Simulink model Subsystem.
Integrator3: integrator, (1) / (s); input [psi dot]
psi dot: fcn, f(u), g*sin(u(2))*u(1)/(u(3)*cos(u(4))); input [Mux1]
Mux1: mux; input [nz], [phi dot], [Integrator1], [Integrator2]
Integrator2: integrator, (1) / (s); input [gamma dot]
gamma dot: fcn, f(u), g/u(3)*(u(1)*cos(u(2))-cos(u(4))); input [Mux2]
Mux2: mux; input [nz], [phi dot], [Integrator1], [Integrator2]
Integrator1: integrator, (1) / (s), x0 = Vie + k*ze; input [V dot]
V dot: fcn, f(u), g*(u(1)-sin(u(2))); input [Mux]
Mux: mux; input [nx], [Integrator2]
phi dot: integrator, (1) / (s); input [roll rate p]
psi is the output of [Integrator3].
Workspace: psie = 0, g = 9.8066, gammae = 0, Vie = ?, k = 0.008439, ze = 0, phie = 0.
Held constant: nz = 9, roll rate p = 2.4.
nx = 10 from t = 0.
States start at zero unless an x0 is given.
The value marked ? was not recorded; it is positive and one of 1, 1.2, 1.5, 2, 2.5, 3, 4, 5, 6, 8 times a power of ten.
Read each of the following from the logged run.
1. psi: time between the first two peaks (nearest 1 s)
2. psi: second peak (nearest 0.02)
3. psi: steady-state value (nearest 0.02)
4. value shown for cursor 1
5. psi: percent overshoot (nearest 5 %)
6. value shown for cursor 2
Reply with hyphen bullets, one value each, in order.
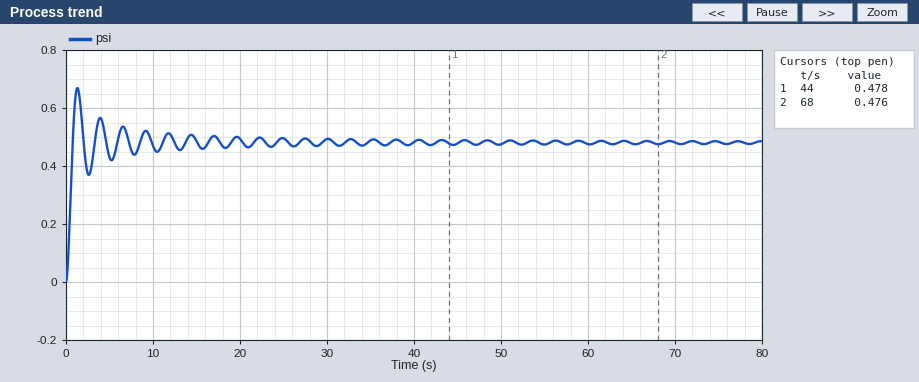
- 3 s
- 0.56
- 0.48
- 0.478
- 40 %
- 0.476
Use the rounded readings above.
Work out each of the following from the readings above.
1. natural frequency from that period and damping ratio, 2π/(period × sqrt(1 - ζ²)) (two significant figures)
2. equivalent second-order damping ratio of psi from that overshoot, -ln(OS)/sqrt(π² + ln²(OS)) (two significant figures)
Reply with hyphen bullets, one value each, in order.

- 2.2 rad/s
- 0.28
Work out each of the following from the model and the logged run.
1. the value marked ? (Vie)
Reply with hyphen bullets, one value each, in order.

- 60
